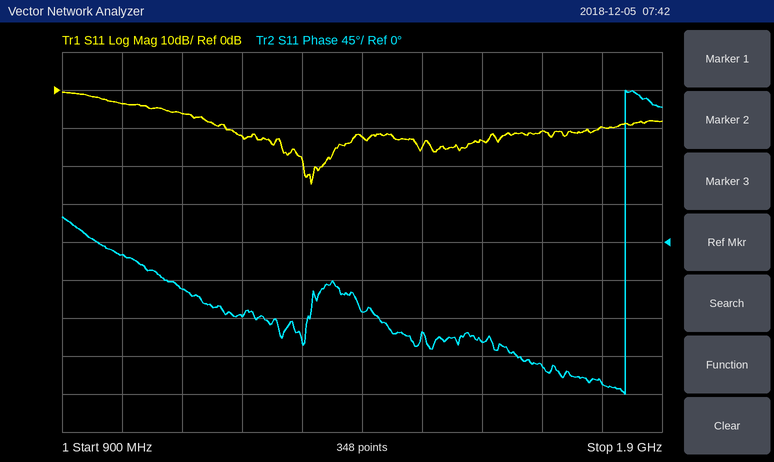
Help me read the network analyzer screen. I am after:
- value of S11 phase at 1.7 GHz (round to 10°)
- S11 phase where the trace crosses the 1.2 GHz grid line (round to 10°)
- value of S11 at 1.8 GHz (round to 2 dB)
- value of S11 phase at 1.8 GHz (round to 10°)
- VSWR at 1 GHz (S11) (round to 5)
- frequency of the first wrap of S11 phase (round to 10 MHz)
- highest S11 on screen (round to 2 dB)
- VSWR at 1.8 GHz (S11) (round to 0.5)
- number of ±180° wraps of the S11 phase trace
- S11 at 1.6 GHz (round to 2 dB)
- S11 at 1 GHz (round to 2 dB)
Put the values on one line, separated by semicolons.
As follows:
-150°; -90°; -10 dB; -170°; 5; 1.84 GHz; 0 dB; 2.0; 1; -14 dB; -4 dB
